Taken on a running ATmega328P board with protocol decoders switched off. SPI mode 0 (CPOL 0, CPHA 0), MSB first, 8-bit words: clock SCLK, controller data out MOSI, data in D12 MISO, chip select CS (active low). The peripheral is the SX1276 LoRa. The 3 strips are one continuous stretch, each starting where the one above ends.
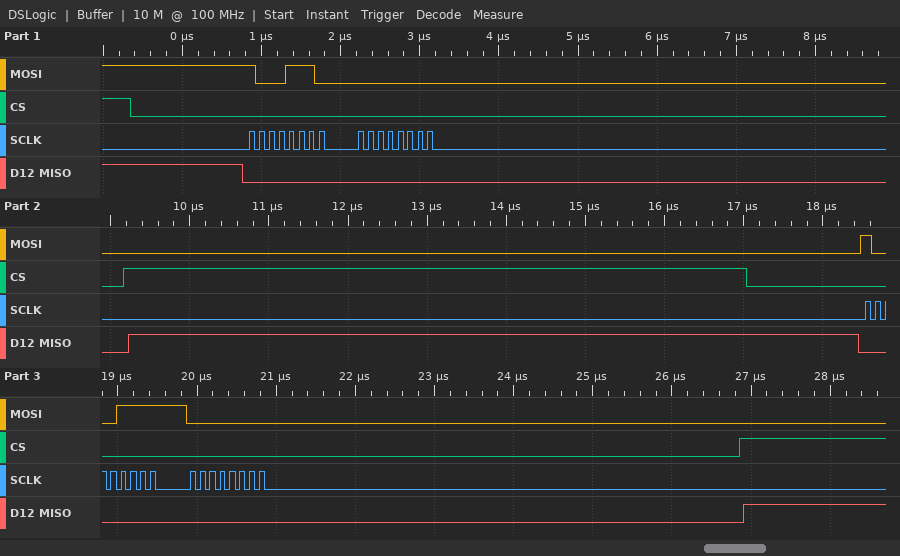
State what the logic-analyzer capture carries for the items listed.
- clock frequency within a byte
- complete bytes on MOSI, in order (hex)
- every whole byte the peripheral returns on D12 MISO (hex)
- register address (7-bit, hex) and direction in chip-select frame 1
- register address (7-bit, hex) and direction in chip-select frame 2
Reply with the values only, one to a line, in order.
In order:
8 MHz
0x8E 0x00 0x8F 0x00
0x00 0x00 0x00 0x00
0x0E write
0x0F write
